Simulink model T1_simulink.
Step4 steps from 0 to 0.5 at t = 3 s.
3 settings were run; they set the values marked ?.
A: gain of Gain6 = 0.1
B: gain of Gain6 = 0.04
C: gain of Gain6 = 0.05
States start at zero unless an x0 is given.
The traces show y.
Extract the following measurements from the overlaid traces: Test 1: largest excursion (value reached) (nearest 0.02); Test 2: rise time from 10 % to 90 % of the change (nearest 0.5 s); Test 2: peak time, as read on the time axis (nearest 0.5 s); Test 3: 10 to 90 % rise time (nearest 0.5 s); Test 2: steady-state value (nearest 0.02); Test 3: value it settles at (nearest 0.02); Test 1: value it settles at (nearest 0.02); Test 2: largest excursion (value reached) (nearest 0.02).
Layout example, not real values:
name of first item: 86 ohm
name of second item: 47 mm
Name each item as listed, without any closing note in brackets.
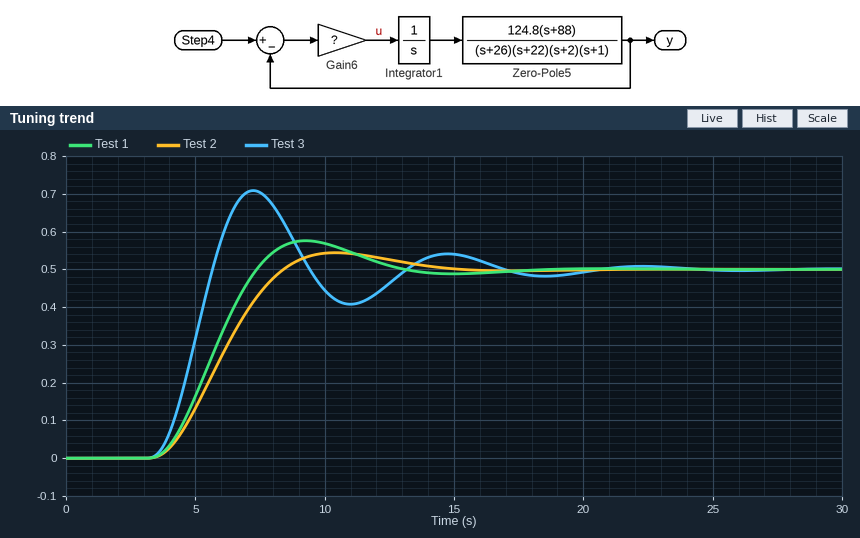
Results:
Test 1: largest excursion (value reached): 0.58
Test 2: rise time from 10 % to 90 % of the change: 3.5 s
Test 2: peak time, as read on the time axis: 10.5 s
Test 3: 10 to 90 % rise time: 1.5 s
Test 2: steady-state value: 0.50
Test 3: value it settles at: 0.50
Test 1: value it settles at: 0.50
Test 2: largest excursion (value reached): 0.54
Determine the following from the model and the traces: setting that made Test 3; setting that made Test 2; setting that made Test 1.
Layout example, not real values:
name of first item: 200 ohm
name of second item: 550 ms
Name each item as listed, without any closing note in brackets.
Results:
setting that made Test 3: A
setting that made Test 2: B
setting that made Test 1: C
